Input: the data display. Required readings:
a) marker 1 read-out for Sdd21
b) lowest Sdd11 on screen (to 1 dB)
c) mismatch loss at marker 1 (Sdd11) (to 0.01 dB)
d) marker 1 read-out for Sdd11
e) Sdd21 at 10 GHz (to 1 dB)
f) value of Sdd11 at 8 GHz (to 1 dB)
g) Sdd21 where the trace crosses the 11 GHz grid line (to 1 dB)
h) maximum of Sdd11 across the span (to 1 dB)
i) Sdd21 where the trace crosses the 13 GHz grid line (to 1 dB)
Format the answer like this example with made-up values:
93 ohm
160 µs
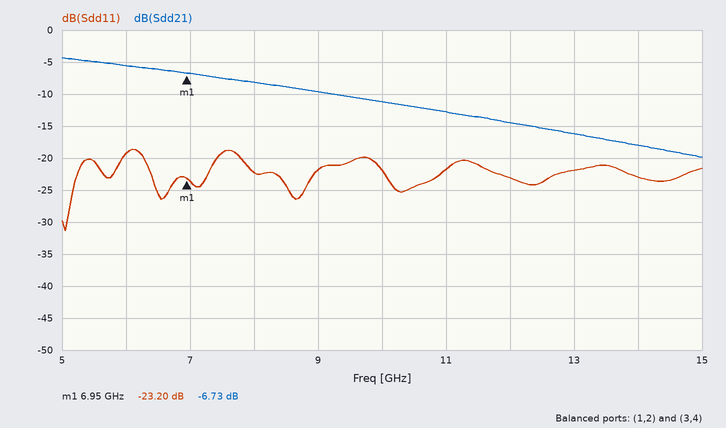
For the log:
-6.73 dB
-31 dB
0.02 dB
-23.20 dB
-11 dB
-22 dB
-13 dB
-19 dB
-16 dB
